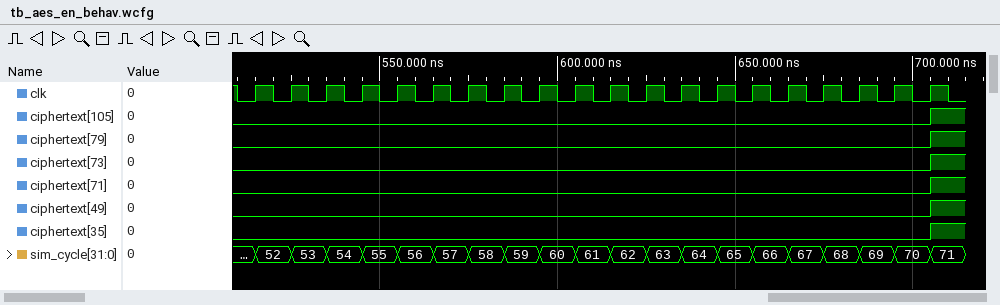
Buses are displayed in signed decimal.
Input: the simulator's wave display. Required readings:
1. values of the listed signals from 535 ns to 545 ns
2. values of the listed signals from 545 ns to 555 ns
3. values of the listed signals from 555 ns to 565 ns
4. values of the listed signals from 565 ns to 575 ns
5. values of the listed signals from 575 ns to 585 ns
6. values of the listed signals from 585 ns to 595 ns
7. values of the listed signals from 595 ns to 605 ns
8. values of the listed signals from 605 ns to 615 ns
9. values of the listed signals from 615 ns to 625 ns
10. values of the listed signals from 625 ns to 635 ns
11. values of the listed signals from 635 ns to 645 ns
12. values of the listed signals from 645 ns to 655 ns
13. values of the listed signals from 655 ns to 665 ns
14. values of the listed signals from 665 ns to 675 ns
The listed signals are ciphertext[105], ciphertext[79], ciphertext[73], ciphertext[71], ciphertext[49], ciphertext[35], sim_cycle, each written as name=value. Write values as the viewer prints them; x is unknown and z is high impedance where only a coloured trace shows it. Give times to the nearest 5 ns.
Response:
ciphertext[105]=0, ciphertext[79]=0, ciphertext[73]=0, ciphertext[71]=0, ciphertext[49]=0, ciphertext[35]=0, sim_cycle=54
ciphertext[105]=0, ciphertext[79]=0, ciphertext[73]=0, ciphertext[71]=0, ciphertext[49]=0, ciphertext[35]=0, sim_cycle=55
ciphertext[105]=0, ciphertext[79]=0, ciphertext[73]=0, ciphertext[71]=0, ciphertext[49]=0, ciphertext[35]=0, sim_cycle=56
ciphertext[105]=0, ciphertext[79]=0, ciphertext[73]=0, ciphertext[71]=0, ciphertext[49]=0, ciphertext[35]=0, sim_cycle=57
ciphertext[105]=0, ciphertext[79]=0, ciphertext[73]=0, ciphertext[71]=0, ciphertext[49]=0, ciphertext[35]=0, sim_cycle=58
ciphertext[105]=0, ciphertext[79]=0, ciphertext[73]=0, ciphertext[71]=0, ciphertext[49]=0, ciphertext[35]=0, sim_cycle=59
ciphertext[105]=0, ciphertext[79]=0, ciphertext[73]=0, ciphertext[71]=0, ciphertext[49]=0, ciphertext[35]=0, sim_cycle=60
ciphertext[105]=0, ciphertext[79]=0, ciphertext[73]=0, ciphertext[71]=0, ciphertext[49]=0, ciphertext[35]=0, sim_cycle=61
ciphertext[105]=0, ciphertext[79]=0, ciphertext[73]=0, ciphertext[71]=0, ciphertext[49]=0, ciphertext[35]=0, sim_cycle=62
ciphertext[105]=0, ciphertext[79]=0, ciphertext[73]=0, ciphertext[71]=0, ciphertext[49]=0, ciphertext[35]=0, sim_cycle=63
ciphertext[105]=0, ciphertext[79]=0, ciphertext[73]=0, ciphertext[71]=0, ciphertext[49]=0, ciphertext[35]=0, sim_cycle=64
ciphertext[105]=0, ciphertext[79]=0, ciphertext[73]=0, ciphertext[71]=0, ciphertext[49]=0, ciphertext[35]=0, sim_cycle=65
ciphertext[105]=0, ciphertext[79]=0, ciphertext[73]=0, ciphertext[71]=0, ciphertext[49]=0, ciphertext[35]=0, sim_cycle=66
ciphertext[105]=0, ciphertext[79]=0, ciphertext[73]=0, ciphertext[71]=0, ciphertext[49]=0, ciphertext[35]=0, sim_cycle=67
